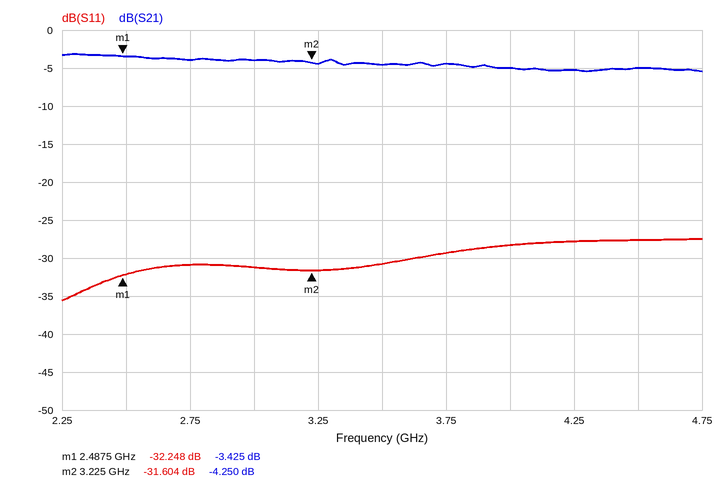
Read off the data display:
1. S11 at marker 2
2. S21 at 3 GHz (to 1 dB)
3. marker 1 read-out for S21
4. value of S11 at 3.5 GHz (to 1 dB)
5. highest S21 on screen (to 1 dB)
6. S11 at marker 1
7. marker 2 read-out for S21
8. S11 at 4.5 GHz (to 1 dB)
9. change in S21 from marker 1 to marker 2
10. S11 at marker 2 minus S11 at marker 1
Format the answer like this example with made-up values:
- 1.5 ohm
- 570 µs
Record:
- -31.604 dB
- -4 dB
- -3.425 dB
- -31 dB
- -3 dB
- -32.248 dB
- -4.250 dB
- -28 dB
- -0.825 dB
- 0.644 dB
